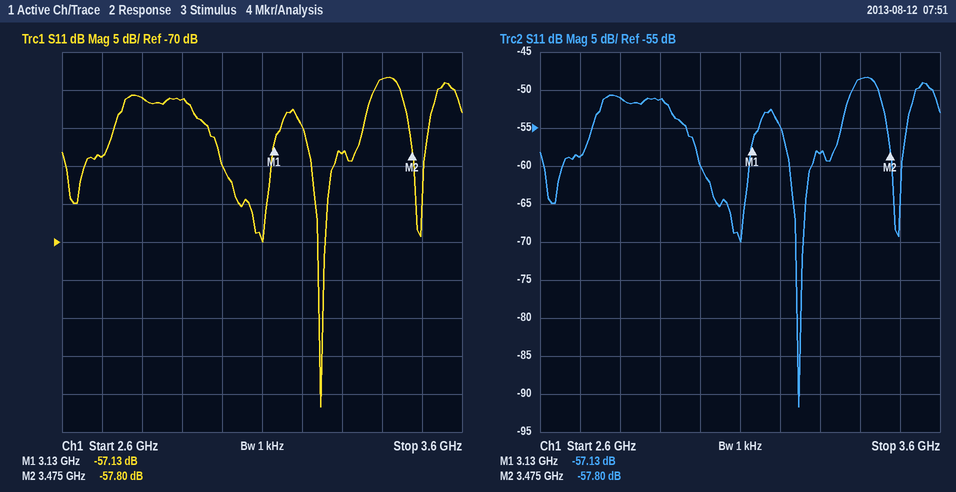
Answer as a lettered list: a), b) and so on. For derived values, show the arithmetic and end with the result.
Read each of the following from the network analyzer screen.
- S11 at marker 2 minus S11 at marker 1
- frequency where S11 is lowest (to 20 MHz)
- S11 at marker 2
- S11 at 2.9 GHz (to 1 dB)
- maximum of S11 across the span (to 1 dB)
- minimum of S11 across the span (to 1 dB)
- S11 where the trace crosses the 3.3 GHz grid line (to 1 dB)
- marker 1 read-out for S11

a) -57.8 − (-57.13) = -0.67 dB
b) 3.24 GHz
c) -57.80 dB
d) -51 dB
e) -48 dB
f) -92 dB
g) -58 dB
h) -57.13 dB
